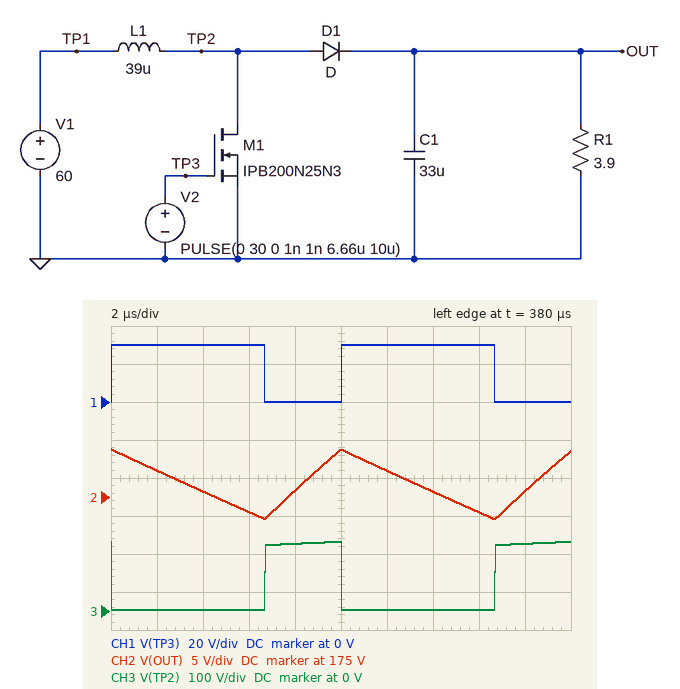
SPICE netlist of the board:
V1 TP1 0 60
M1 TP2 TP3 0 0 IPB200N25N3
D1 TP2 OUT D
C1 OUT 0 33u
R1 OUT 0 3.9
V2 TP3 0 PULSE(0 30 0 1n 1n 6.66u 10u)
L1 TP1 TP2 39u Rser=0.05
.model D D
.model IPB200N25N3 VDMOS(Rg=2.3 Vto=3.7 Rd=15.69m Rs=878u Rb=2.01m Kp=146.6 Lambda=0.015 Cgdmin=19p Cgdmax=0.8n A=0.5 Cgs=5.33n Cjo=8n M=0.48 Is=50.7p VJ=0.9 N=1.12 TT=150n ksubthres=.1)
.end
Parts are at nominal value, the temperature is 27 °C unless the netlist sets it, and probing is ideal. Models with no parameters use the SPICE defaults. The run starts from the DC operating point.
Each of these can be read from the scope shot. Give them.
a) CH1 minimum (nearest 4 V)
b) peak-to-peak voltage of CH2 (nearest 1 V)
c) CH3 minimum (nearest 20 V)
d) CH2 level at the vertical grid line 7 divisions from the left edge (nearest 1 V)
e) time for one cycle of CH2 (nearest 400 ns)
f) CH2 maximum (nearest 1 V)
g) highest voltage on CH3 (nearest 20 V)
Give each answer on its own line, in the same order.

0 V
9 V
0 V
176 V
10.0 µs
181 V
180 V
